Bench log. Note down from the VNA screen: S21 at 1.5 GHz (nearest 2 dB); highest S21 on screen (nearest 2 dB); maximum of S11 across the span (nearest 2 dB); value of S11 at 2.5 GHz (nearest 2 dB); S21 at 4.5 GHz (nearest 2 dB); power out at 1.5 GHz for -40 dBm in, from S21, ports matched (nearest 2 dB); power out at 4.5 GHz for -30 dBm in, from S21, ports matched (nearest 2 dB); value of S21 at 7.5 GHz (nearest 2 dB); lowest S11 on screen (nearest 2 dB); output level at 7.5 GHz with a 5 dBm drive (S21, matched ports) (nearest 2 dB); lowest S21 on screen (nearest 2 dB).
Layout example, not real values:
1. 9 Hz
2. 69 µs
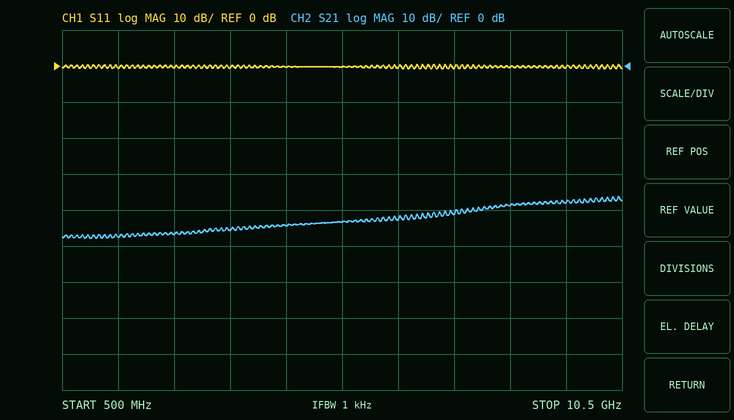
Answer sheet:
1. -48 dB
2. -36 dB
3. 0 dB
4. 0 dB
5. -44 dB
6. -88 dBm
7. -74 dBm
8. -42 dB
9. 0 dB
10. -36 dBm
11. -48 dB
